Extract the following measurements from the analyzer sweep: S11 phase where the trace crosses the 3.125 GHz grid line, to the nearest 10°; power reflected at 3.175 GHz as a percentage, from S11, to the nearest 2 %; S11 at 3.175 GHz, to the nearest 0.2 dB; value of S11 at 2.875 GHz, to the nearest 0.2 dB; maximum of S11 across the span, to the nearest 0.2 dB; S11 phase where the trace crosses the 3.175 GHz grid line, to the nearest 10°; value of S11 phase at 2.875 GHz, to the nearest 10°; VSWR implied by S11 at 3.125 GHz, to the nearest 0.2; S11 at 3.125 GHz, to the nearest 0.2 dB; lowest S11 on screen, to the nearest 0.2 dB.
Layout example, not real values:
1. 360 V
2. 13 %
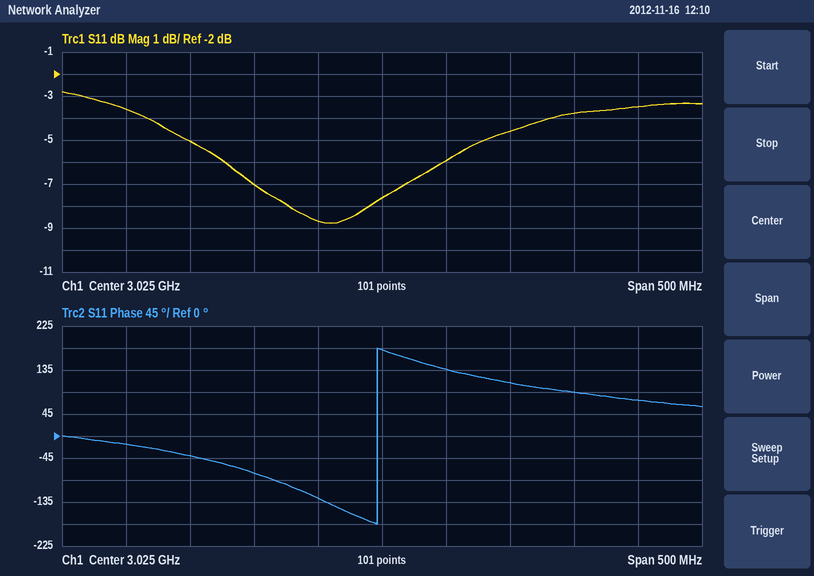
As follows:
1. 110°
2. 42 %
3. -3.8 dB
4. -5.0 dB
5. -2.8 dB
6. 90°
7. -40°
8. 3.8
9. -4.6 dB
10. -8.8 dB
